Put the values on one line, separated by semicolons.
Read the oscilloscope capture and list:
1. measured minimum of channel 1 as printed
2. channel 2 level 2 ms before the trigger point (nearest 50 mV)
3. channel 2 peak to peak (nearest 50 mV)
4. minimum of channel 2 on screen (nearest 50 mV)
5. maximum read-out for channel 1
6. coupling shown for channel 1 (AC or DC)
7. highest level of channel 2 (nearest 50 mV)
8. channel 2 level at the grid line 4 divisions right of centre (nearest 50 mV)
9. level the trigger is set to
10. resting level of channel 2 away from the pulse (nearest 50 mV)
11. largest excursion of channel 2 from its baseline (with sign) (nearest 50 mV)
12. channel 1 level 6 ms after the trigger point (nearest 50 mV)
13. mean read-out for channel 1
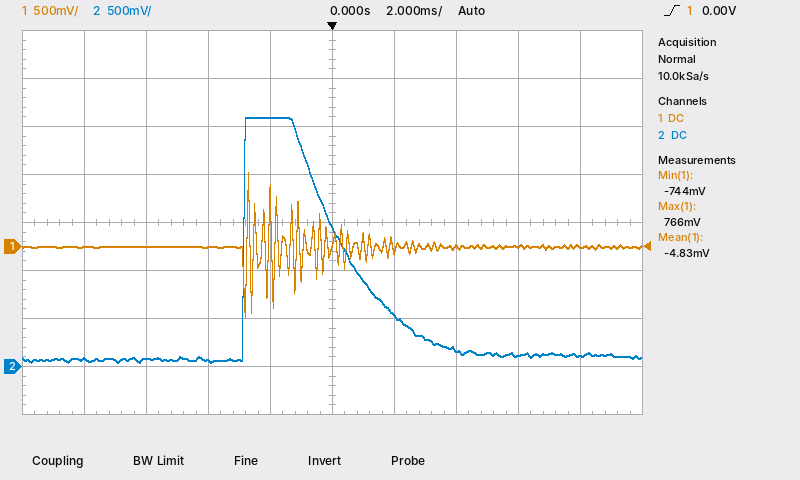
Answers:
-744 mV; 2.60 V; 2.55 V; 50 mV; 766 mV; DC; 2.60 V; 100 mV; 0.00 V; 100 mV; +2.50 V; 0 mV; -4.83 mV
